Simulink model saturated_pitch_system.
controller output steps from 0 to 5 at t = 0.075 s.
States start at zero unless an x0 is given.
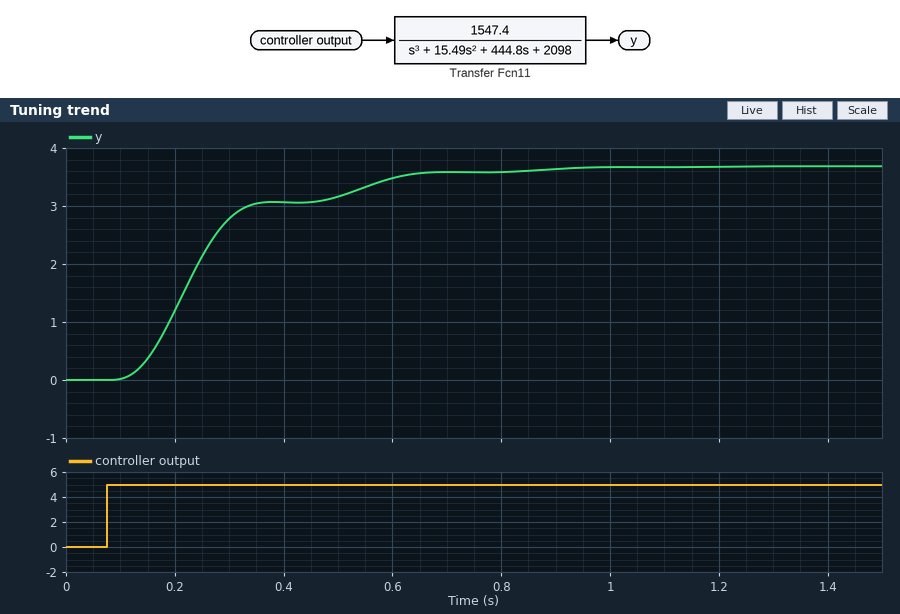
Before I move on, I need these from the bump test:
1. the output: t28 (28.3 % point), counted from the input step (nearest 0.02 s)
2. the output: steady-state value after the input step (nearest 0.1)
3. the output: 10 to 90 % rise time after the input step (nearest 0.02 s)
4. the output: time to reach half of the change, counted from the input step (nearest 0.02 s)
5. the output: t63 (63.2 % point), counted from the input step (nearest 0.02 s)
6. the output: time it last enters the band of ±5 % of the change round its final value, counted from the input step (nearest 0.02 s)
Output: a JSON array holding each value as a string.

["0.12 s", "3.7", "0.40 s", "0.16 s", "0.18 s", "0.54 s"]
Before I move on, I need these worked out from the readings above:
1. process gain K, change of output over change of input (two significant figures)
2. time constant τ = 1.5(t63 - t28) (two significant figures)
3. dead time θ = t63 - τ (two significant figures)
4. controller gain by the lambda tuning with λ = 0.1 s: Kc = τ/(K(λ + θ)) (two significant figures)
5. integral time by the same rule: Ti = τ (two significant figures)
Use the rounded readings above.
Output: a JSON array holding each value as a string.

["0.74", "0.090 s", "0.090 s", "0.64", "0.090 s"]
